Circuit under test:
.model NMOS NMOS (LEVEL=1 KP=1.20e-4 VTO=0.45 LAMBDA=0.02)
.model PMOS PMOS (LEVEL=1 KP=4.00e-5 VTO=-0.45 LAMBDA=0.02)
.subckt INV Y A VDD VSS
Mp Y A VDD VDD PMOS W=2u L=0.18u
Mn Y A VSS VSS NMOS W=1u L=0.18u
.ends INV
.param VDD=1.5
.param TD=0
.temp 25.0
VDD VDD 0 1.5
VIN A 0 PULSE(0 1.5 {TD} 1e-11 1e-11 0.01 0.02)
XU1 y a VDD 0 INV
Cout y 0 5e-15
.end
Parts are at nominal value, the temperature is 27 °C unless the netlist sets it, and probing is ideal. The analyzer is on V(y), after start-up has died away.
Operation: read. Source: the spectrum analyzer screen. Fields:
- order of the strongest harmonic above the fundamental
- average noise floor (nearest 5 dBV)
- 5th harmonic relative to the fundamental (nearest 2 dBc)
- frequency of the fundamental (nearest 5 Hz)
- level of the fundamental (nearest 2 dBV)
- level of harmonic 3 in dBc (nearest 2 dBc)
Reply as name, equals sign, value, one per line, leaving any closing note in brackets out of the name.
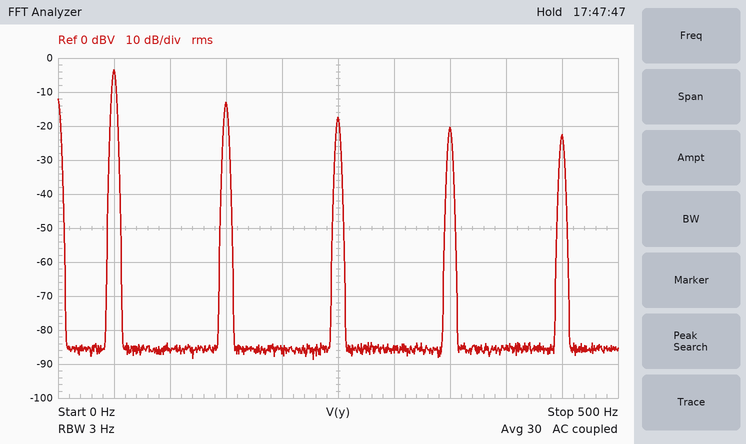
order of the strongest harmonic above the fundamental = 3
average noise floor = -85 dBV
5th harmonic relative to the fundamental = -14 dBc
frequency of the fundamental = 50 Hz
level of the fundamental = -4 dBV
level of harmonic 3 in dBc = -10 dBc
